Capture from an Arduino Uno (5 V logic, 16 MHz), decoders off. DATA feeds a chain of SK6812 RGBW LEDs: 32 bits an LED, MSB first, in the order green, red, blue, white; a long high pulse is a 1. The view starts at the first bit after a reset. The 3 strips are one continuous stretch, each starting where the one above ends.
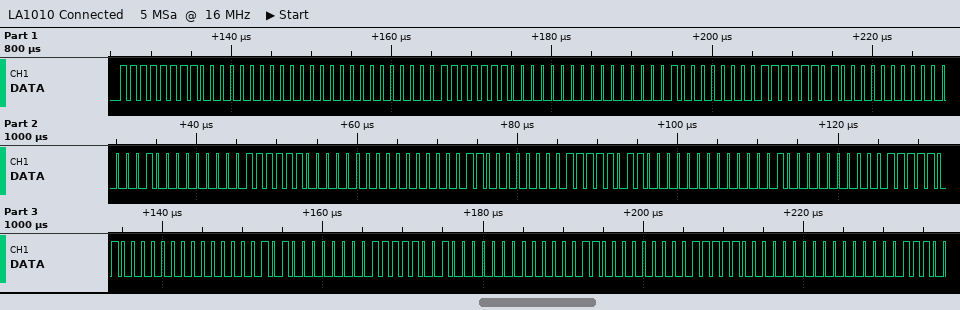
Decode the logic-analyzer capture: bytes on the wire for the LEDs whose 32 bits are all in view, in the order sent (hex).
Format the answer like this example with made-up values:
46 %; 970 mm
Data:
FF 00 00 00 FE 00 01 00 FD 00 02 00 FC 00 03 00 FB 00 04 00 FA 00 05 00 F9 00 06 00
